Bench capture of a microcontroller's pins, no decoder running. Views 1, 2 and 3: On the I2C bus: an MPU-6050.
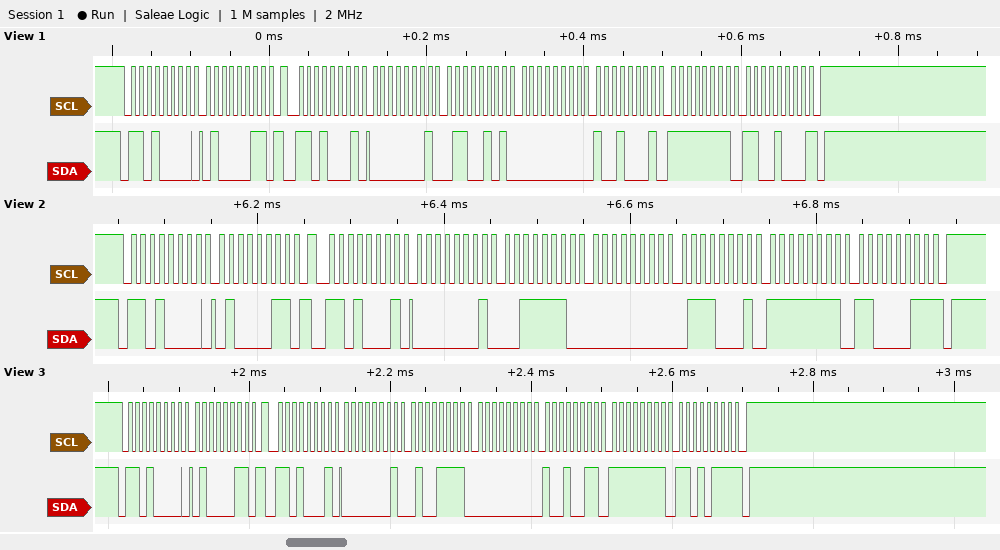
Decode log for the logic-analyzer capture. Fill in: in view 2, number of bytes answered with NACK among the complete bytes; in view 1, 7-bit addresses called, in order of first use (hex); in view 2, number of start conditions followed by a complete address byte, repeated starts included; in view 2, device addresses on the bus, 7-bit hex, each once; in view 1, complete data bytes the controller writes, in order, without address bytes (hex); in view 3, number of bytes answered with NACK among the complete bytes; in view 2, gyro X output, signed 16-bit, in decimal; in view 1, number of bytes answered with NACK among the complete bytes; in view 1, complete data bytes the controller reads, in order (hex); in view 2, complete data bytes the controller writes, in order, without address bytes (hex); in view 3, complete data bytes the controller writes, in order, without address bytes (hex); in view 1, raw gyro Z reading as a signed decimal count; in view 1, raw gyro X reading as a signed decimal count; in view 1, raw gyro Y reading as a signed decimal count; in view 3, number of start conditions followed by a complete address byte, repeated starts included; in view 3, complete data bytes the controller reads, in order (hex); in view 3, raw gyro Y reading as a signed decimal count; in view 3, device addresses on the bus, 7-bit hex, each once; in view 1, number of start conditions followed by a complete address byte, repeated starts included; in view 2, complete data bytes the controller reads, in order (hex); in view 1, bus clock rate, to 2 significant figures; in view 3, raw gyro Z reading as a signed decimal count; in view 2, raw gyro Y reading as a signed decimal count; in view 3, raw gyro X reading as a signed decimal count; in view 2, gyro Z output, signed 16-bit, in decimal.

1
0x68
2
0x68
43
1
318
1
01 65 00 91 FF C8
43
43
-56
357
145
2
01 4F 00 93 FF D7
147
0x68
2
01 3E 00 71 FF C3
100 kHz
-41
113
335
-61
